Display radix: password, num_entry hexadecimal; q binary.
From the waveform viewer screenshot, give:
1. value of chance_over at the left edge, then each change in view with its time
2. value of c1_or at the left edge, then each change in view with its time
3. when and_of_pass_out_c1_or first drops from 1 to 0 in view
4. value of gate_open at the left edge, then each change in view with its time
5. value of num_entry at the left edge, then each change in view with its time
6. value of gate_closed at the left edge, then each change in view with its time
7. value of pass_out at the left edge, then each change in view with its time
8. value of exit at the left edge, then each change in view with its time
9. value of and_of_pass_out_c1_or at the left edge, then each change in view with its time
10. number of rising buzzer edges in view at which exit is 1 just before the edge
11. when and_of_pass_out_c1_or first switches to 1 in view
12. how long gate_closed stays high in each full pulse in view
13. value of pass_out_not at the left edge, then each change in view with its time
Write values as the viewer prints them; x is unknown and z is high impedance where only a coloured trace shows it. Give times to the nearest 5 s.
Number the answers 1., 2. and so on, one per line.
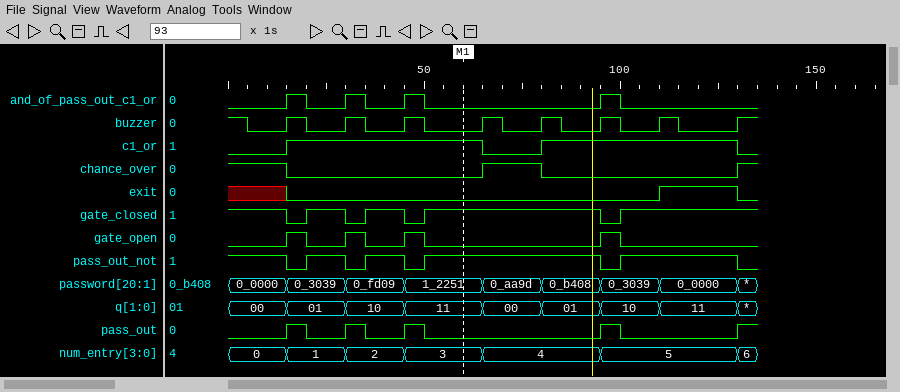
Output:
1. 1, 0 at 15 s, 1 at 65 s, 0 at 80 s, 1 at 130 s
2. 0, 1 at 15 s, 0 at 65 s, 1 at 80 s, 0 at 130 s
3. 20 s
4. 0, 1 at 15 s, 0 at 20 s, 1 at 30 s, 0 at 35 s, 1 at 45 s, 0 at 50 s, 1 at 95 s, 0 at 100 s
5. 0, 1 at 15 s, 2 at 30 s, 3 at 45 s, 4 at 65 s, 5 at 95 s, 6 at 130 s
6. 1, 0 at 15 s, 1 at 20 s, 0 at 30 s, 1 at 35 s, 0 at 45 s, 1 at 50 s, 0 at 95 s, 1 at 100 s
7. 0, 1 at 15 s, 0 at 20 s, 1 at 30 s, 0 at 35 s, 1 at 45 s, 0 at 50 s, 1 at 95 s, 0 at 100 s, 1 at 130 s
8. x, 0 at 15 s, 1 at 110 s, 0 at 130 s
9. 0, 1 at 15 s, 0 at 20 s, 1 at 30 s, 0 at 35 s, 1 at 45 s, 0 at 50 s, 1 at 95 s, 0 at 100 s
10. 1
11. 15 s
12. 10 s, 10 s, 45 s
13. 1, 0 at 15 s, 1 at 20 s, 0 at 30 s, 1 at 35 s, 0 at 45 s, 1 at 50 s, 0 at 95 s, 1 at 100 s, 0 at 130 s
